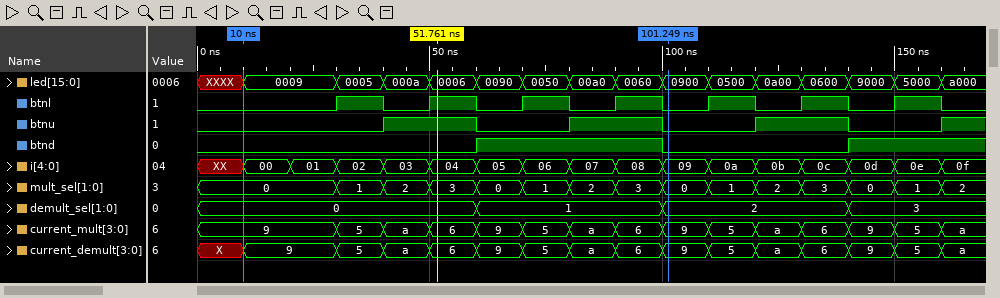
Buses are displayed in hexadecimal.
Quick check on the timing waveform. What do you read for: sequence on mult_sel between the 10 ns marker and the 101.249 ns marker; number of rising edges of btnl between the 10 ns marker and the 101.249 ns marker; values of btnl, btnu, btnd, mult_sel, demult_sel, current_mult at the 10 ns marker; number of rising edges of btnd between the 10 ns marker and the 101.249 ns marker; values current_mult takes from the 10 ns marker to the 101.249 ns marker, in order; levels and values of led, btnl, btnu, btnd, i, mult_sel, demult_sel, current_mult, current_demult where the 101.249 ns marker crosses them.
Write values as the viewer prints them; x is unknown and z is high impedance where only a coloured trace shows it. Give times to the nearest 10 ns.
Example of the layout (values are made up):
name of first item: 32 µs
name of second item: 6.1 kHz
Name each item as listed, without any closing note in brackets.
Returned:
sequence on mult_sel between the 10 ns marker and the 101.249 ns marker: 0, 1, 2, 3, 0, 1, 2, 3, 0
number of rising edges of btnl between the 10 ns marker and the 101.249 ns marker: 4
values of btnl, btnu, btnd, mult_sel, demult_sel, current_mult at the 10 ns marker: btnl=0, btnu=0, btnd=0, mult_sel=0, demult_sel=0, current_mult=9
number of rising edges of btnd between the 10 ns marker and the 101.249 ns marker: 1
values current_mult takes from the 10 ns marker to the 101.249 ns marker, in order: 9, 5, a, 6, 9, 5, a, 6, 9
levels and values of led, btnl, btnu, btnd, i, mult_sel, demult_sel, current_mult, current_demult where the 101.249 ns marker crosses them: led=0900, btnl=0, btnu=0, btnd=0, i=09, mult_sel=0, demult_sel=2, current_mult=9, current_demult=9
